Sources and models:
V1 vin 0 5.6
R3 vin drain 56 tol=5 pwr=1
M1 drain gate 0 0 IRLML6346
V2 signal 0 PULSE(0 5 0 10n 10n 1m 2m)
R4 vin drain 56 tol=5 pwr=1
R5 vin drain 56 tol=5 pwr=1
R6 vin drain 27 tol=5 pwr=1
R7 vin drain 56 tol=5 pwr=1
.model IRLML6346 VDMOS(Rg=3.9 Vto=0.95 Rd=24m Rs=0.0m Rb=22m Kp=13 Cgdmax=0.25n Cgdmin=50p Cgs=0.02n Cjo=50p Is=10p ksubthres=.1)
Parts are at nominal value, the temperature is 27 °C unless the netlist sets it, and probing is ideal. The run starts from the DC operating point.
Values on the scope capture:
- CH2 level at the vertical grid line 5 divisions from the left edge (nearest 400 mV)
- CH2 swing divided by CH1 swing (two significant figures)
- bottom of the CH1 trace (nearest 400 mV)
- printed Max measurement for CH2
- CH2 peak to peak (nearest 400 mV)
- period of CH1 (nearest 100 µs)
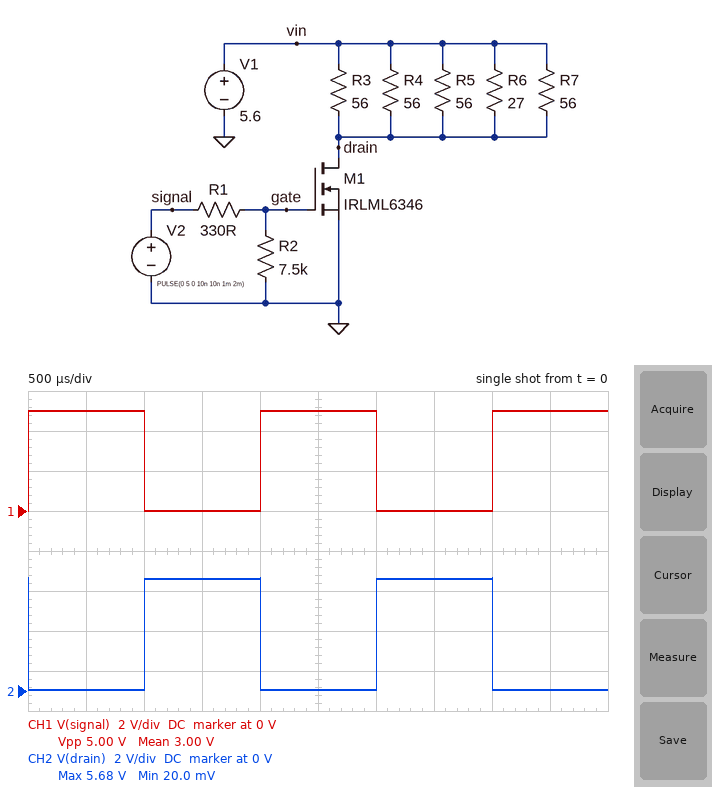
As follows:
0 V
1.1
0 V
5.68 V
5.6 V
2.0 ms
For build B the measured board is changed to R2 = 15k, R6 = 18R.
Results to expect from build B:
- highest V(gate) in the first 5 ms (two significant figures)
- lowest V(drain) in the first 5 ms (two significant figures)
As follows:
4.9 V
31 mV
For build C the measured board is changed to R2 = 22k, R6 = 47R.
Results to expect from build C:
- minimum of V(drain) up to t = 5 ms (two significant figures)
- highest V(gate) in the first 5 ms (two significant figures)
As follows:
22 mV
4.9 V
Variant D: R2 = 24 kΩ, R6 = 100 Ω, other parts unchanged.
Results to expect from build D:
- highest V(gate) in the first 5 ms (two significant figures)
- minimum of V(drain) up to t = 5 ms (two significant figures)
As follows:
4.9 V
20 mV
